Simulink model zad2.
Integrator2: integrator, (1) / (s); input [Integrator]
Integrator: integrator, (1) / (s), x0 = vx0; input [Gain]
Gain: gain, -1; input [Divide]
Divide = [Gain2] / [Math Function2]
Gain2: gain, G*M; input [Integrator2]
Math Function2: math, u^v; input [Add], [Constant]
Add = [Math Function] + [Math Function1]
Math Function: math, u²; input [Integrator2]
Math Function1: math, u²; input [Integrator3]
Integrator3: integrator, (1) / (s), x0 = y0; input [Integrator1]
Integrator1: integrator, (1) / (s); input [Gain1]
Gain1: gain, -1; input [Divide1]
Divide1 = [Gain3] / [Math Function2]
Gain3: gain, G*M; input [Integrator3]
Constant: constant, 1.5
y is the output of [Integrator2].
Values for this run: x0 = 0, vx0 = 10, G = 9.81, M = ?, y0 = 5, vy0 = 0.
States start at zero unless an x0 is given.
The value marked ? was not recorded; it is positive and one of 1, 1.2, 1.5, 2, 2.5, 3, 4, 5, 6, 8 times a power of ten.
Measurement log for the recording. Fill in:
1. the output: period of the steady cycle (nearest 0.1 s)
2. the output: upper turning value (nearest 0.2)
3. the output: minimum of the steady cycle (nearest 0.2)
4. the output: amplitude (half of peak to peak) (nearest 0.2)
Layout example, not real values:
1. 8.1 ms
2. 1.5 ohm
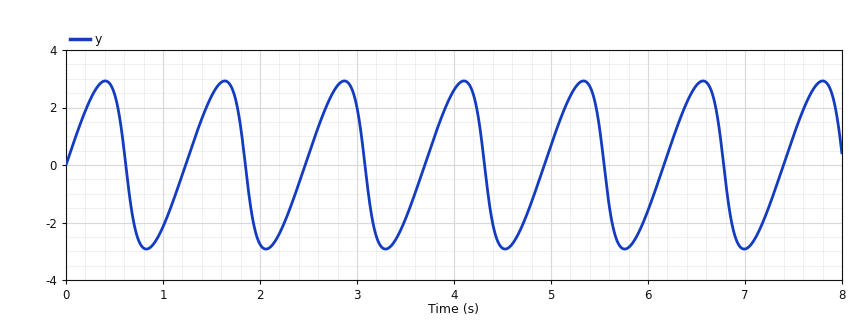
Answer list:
1. 1.2 s
2. 3.0
3. -3.0
4. 3.0
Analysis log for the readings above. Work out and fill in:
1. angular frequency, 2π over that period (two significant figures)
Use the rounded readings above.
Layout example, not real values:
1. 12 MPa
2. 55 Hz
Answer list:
1. 5.2 rad/s
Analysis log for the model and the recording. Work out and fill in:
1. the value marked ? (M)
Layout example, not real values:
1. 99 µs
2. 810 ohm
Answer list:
1. 100
